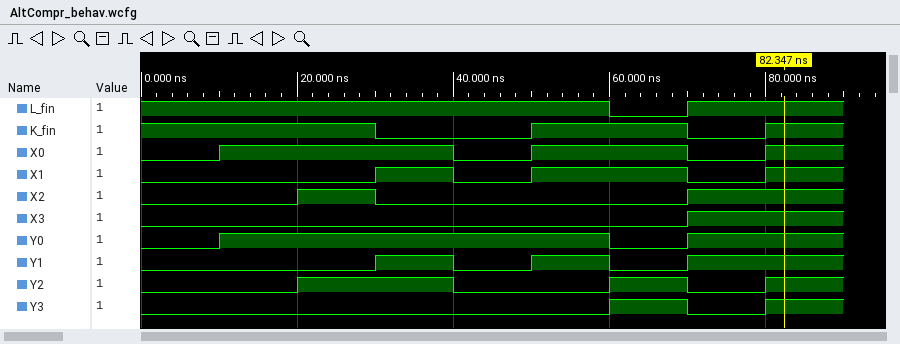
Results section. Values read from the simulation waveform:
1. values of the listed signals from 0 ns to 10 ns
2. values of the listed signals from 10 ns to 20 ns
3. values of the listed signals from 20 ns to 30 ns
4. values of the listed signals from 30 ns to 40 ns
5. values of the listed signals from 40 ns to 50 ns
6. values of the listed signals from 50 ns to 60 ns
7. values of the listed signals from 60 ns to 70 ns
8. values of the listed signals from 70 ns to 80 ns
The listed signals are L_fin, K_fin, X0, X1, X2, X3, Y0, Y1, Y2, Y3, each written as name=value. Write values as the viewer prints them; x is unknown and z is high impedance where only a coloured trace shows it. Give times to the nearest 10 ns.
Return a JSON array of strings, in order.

["L_fin=1, K_fin=1, X0=0, X1=0, X2=0, X3=0, Y0=0, Y1=0, Y2=0, Y3=0", "L_fin=1, K_fin=1, X0=1, X1=0, X2=0, X3=0, Y0=1, Y1=0, Y2=0, Y3=0", "L_fin=1, K_fin=1, X0=1, X1=0, X2=1, X3=0, Y0=1, Y1=0, Y2=1, Y3=0", "L_fin=1, K_fin=0, X0=1, X1=1, X2=0, X3=0, Y0=1, Y1=1, Y2=1, Y3=0", "L_fin=1, K_fin=0, X0=0, X1=0, X2=0, X3=0, Y0=1, Y1=0, Y2=0, Y3=0", "L_fin=1, K_fin=1, X0=1, X1=1, X2=0, X3=0, Y0=1, Y1=1, Y2=0, Y3=0", "L_fin=0, K_fin=1, X0=1, X1=1, X2=0, X3=0, Y0=0, Y1=0, Y2=1, Y3=1", "L_fin=1, K_fin=0, X0=0, X1=0, X2=1, X3=1, Y0=1, Y1=1, Y2=0, Y3=0"]
